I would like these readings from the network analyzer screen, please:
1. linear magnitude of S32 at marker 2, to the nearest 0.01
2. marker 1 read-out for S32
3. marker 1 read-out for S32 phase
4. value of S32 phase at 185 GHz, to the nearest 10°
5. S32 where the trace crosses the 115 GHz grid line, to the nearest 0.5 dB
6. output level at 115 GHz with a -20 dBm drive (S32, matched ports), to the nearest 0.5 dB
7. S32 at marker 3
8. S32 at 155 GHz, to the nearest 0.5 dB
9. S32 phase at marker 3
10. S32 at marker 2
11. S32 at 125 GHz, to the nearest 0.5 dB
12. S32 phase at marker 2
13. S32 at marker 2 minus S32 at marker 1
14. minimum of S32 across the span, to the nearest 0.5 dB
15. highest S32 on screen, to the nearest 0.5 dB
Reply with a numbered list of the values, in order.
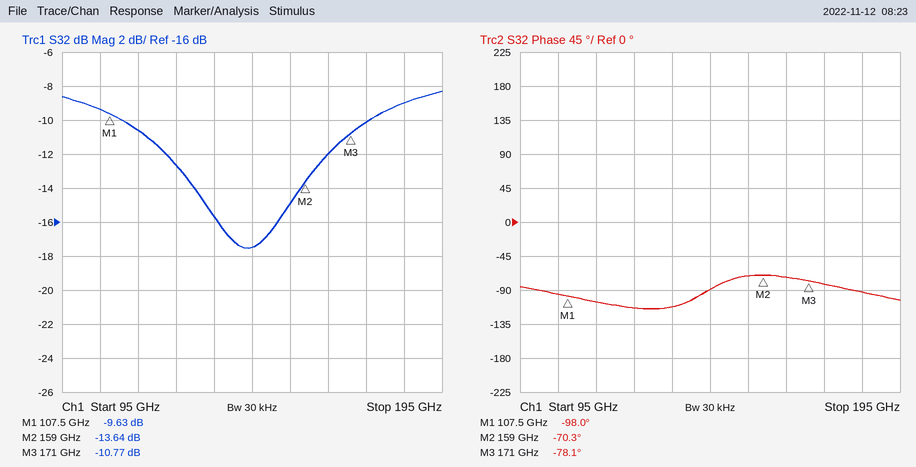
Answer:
1. 0.21
2. -9.63 dB
3. -98.0°
4. -90°
5. -10.5 dB
6. -30.5 dBm
7. -10.77 dB
8. -15.0 dB
9. -78.1°
10. -13.64 dB
11. -12.5 dB
12. -70.3°
13. -4.01 dB
14. -17.5 dB
15. -8.5 dB
